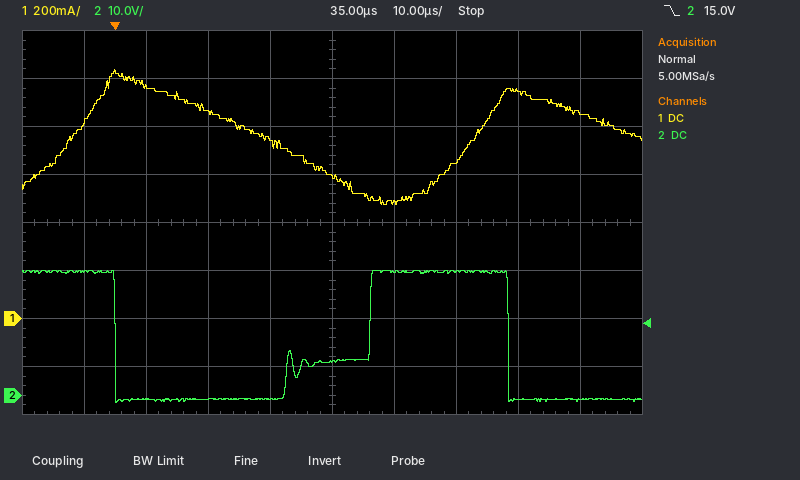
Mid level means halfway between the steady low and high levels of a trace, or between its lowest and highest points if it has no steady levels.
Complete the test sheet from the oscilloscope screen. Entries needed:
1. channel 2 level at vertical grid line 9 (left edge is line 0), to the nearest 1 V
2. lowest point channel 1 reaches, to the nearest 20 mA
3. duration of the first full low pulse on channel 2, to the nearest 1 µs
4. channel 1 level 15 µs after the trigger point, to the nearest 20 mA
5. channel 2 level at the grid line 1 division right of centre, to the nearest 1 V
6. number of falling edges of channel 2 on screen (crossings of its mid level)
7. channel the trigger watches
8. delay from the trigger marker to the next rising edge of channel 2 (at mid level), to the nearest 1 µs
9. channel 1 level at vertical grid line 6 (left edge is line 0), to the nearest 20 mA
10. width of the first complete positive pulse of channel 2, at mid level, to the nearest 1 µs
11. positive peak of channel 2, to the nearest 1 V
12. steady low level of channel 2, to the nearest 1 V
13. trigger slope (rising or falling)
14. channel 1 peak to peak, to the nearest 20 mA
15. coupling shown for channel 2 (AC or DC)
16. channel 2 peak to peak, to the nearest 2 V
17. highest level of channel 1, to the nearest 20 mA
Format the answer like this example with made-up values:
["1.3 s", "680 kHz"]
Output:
["-1 V", "480 mA", "41 µs", "860 mA", "26 V", "2", "channel 2", "41 µs", "480 mA", "22 µs", "26 V", "-1 V", "falling", "560 mA", "DC", "28 V", "1.04 A"]
